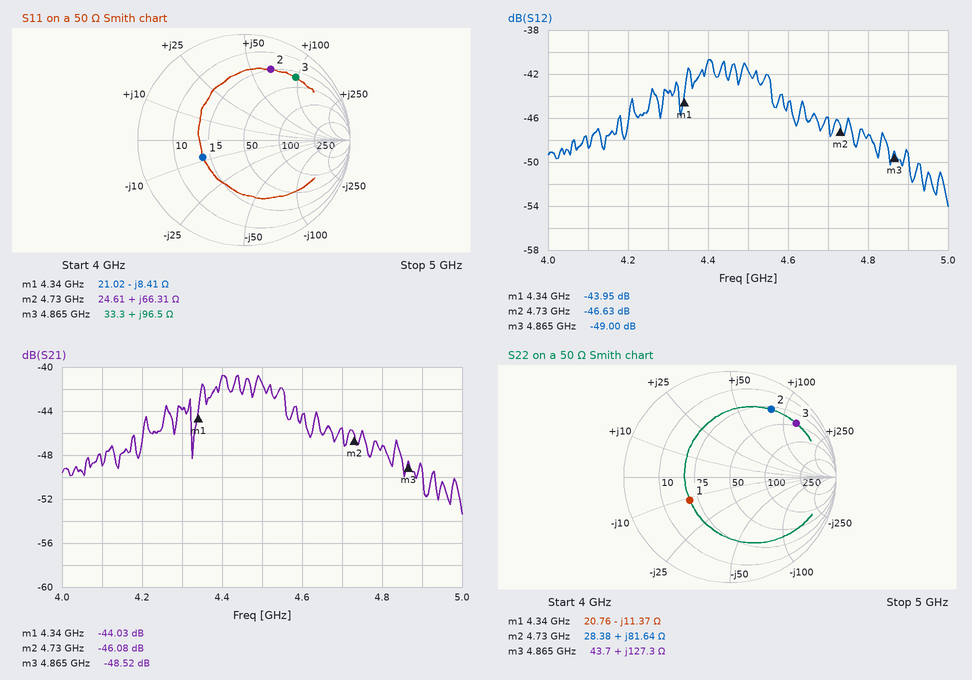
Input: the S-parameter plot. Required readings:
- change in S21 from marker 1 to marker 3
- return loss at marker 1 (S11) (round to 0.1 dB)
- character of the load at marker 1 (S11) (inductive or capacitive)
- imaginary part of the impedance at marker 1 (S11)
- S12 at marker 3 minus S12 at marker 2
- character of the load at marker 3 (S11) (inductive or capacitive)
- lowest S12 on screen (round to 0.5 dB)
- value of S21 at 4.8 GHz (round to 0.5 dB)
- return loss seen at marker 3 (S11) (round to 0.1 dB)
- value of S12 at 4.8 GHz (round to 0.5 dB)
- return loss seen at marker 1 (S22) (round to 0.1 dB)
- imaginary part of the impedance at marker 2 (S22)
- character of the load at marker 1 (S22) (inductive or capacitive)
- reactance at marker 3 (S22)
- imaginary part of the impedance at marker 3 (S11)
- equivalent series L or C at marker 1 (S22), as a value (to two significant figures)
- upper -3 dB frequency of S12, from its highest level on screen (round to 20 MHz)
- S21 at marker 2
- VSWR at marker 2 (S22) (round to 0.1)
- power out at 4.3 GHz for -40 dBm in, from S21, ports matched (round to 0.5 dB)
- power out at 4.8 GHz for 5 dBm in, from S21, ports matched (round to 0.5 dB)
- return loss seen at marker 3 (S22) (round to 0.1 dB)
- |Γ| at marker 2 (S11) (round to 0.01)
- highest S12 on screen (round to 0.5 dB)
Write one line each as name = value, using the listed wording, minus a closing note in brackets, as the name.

change in S21 from marker 1 to marker 3 = -4.49 dB
return loss at marker 1 (S11) = 7.5 dB
character of the load at marker 1 (S11) = capacitive
imaginary part of the impedance at marker 1 = -8.41 Ω
S12 at marker 3 minus S12 at marker 2 = -2.37 dB
character of the load at marker 3 (S11) = inductive
lowest S12 on screen = -54.0 dB
value of S21 at 4.8 GHz = -47.0 dB
return loss seen at marker 3 (S11) = 2.3 dB
value of S12 at 4.8 GHz = -47.5 dB
return loss seen at marker 1 (S22) = 7.2 dB
imaginary part of the impedance at marker 2 = +81.64 Ω
character of the load at marker 1 (S22) = capacitive
reactance at marker 3 = +127.3 Ω
imaginary part of the impedance at marker 3 = +96.5 Ω
equivalent series L or C at marker 1 (S22), as a value = 3.2 pF
upper -3 dB frequency of S12, from its highest level on screen = 4.56 GHz
S21 at marker 2 = -46.08 dB
VSWR at marker 2 (S22) = 6.9
power out at 4.3 GHz for -40 dBm in, from S21, ports matched = -84.0 dBm
power out at 4.8 GHz for 5 dBm in, from S21, ports matched = -42.0 dBm
return loss seen at marker 3 (S22) = 1.9 dB
|Γ| at marker 2 (S11) = 0.71
highest S12 on screen = -40.5 dB
